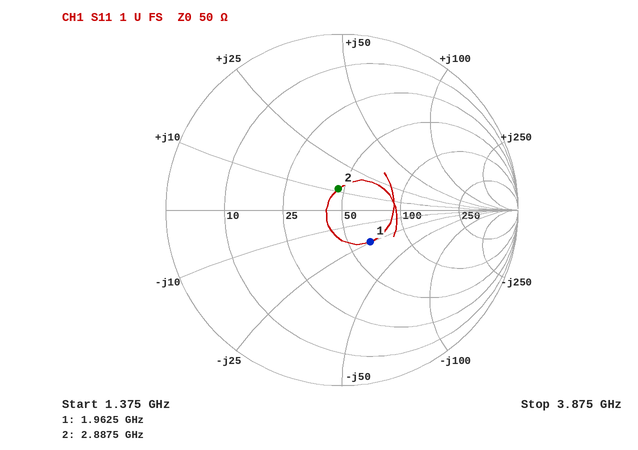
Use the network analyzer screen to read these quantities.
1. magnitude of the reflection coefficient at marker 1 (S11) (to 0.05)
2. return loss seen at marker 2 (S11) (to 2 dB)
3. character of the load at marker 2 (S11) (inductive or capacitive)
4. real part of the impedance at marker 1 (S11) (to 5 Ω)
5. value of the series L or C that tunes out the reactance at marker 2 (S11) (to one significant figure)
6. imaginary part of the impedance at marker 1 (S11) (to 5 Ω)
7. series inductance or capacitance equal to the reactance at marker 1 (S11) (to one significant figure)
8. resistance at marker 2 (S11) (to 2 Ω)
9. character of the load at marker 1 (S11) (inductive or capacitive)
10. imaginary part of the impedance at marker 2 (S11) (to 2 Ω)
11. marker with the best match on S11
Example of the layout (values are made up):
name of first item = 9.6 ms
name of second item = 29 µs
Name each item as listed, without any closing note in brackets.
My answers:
magnitude of the reflection coefficient at marker 1 (S11) = 0.25
return loss seen at marker 2 (S11) = 18 dB
character of the load at marker 2 (S11) = inductive
real part of the impedance at marker 1 (S11) = 65 Ω
value of the series L or C that tunes out the reactance at marker 2 (S11) = 5 pF
imaginary part of the impedance at marker 1 (S11) = -25 Ω
series inductance or capacitance equal to the reactance at marker 1 (S11) = 3 pF
resistance at marker 2 (S11) = 46 Ω
character of the load at marker 1 (S11) = capacitive
imaginary part of the impedance at marker 2 (S11) = +12 Ω
marker with the best match on S11 = marker 2
